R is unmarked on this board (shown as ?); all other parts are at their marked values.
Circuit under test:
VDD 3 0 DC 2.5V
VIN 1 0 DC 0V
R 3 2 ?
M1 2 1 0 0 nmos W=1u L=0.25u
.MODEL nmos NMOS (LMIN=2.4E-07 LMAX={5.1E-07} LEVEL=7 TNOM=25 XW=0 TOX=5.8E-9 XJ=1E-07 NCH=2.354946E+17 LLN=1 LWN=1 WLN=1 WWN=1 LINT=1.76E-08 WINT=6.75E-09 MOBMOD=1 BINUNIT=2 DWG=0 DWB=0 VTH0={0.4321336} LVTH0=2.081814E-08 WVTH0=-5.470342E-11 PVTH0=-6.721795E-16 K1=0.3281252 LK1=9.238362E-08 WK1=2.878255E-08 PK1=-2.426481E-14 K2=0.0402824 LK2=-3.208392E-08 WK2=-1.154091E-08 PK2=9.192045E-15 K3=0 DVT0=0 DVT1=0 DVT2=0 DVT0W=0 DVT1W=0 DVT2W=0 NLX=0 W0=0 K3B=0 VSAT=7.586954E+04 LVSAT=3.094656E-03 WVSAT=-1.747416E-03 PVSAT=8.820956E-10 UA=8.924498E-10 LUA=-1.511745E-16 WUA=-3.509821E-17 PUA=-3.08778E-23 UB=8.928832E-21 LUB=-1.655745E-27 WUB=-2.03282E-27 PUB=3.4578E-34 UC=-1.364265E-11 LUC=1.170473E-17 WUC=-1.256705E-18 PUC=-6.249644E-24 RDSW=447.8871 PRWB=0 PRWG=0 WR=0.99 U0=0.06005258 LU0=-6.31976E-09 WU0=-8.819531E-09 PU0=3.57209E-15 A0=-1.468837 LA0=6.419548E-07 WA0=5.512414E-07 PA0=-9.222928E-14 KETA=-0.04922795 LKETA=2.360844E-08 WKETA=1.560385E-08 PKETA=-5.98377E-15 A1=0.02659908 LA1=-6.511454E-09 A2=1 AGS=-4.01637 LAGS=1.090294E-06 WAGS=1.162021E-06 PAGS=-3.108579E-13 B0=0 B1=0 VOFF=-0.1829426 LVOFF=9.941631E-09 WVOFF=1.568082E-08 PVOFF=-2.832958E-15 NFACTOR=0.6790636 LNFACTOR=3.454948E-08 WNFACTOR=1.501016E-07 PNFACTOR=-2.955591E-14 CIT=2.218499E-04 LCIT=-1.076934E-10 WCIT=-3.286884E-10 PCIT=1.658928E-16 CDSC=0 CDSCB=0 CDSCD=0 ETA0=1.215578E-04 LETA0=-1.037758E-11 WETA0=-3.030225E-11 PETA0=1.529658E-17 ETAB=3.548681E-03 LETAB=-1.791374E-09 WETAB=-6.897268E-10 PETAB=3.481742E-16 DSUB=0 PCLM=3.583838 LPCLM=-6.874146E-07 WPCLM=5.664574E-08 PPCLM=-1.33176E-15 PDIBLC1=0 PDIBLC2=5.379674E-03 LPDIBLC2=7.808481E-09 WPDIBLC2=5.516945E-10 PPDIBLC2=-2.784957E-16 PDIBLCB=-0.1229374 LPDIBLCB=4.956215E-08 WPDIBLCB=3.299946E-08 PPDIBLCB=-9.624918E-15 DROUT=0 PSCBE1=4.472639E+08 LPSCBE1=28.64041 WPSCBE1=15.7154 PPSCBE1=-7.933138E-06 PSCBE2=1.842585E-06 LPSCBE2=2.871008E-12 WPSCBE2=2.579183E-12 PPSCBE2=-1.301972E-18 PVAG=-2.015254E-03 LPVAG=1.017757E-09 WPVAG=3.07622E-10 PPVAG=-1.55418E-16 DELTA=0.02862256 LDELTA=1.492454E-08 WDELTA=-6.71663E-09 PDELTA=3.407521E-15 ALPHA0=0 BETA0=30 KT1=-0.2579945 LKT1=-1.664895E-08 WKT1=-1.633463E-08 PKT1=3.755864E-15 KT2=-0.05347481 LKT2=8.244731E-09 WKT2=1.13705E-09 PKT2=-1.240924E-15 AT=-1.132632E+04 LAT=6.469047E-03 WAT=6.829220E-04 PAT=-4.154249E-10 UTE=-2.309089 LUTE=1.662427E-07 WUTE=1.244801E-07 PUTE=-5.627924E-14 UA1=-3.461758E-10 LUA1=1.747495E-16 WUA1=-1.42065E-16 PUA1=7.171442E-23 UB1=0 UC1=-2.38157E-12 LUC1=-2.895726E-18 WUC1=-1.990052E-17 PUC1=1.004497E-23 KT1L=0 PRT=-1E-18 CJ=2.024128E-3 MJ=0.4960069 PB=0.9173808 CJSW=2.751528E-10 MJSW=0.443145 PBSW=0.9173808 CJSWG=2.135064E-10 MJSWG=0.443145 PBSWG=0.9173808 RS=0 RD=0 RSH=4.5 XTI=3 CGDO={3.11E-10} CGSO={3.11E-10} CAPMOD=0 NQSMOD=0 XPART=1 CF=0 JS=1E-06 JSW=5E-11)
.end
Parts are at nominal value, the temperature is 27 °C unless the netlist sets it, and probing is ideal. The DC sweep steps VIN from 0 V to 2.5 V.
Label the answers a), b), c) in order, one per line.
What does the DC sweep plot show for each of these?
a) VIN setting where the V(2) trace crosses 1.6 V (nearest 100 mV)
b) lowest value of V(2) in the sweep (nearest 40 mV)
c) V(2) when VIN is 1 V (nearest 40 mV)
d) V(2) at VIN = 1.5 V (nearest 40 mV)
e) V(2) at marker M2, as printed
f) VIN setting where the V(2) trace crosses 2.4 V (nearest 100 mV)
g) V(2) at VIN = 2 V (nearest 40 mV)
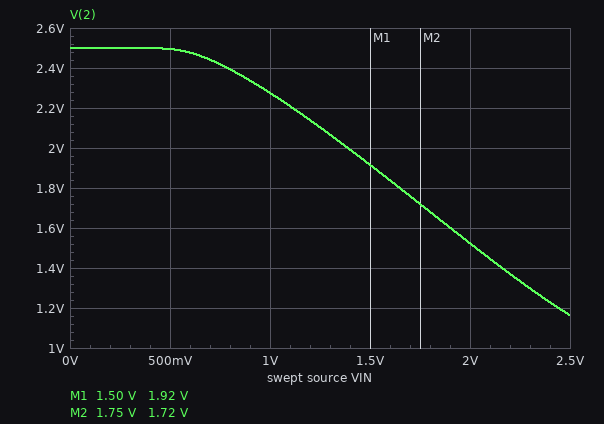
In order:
a) 1.9 V
b) 1.16 V
c) 2.28 V
d) 1.92 V
e) 1.72 V
f) 800 mV
g) 1.52 V
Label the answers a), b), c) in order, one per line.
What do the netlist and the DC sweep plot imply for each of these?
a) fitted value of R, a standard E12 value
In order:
a) 2.7 kΩ
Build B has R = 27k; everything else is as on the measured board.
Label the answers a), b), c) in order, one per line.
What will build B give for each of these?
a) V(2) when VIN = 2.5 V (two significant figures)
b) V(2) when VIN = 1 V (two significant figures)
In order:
a) 100 mV
b) 700 mV
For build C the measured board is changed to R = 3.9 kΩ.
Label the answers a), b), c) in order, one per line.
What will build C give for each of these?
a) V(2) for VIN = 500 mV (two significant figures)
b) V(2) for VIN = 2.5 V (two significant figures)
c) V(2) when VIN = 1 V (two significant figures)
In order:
a) 2.5 V
b) 800 mV
c) 2.2 V
